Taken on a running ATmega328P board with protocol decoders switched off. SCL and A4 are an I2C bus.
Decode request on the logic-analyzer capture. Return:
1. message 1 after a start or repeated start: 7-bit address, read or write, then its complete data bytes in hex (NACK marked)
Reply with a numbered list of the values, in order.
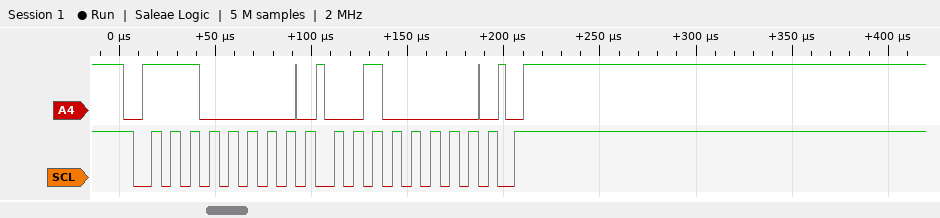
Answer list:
1. 0x70 write: 20
